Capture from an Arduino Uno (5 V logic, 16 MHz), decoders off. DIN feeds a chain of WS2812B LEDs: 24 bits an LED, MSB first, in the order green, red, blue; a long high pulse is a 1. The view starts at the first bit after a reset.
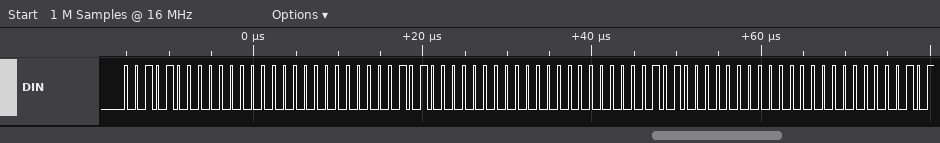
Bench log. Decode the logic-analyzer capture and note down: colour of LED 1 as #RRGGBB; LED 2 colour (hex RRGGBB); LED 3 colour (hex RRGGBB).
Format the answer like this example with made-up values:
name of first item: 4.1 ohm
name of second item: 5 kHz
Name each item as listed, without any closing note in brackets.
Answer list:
colour of LED 1 as #RRGGBB: #002800
LED 2 colour: #002800
LED 3 colour: #002800
